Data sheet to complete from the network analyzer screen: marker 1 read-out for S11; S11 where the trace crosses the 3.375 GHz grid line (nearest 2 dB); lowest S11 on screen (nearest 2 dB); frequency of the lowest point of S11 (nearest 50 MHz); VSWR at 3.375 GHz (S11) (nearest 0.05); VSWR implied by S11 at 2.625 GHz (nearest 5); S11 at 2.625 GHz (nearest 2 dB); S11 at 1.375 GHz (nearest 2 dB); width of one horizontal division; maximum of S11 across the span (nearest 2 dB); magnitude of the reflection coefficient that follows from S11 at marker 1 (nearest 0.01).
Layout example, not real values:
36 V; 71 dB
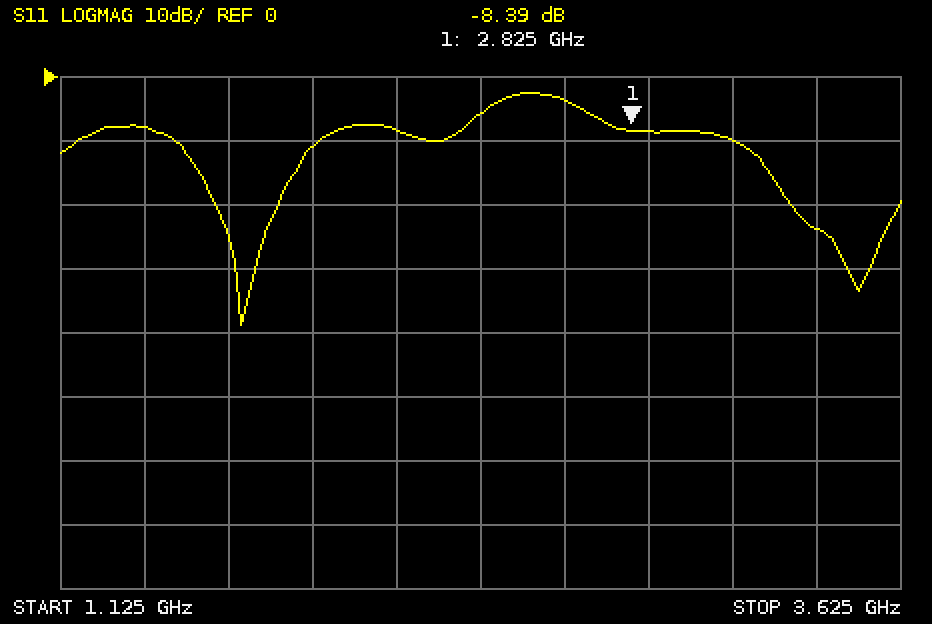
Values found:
-8.39 dB; -24 dB; -38 dB; 1.65 GHz; 1.15; 5; -4 dB; -8 dB; 250 MHz; -2 dB; 0.38
